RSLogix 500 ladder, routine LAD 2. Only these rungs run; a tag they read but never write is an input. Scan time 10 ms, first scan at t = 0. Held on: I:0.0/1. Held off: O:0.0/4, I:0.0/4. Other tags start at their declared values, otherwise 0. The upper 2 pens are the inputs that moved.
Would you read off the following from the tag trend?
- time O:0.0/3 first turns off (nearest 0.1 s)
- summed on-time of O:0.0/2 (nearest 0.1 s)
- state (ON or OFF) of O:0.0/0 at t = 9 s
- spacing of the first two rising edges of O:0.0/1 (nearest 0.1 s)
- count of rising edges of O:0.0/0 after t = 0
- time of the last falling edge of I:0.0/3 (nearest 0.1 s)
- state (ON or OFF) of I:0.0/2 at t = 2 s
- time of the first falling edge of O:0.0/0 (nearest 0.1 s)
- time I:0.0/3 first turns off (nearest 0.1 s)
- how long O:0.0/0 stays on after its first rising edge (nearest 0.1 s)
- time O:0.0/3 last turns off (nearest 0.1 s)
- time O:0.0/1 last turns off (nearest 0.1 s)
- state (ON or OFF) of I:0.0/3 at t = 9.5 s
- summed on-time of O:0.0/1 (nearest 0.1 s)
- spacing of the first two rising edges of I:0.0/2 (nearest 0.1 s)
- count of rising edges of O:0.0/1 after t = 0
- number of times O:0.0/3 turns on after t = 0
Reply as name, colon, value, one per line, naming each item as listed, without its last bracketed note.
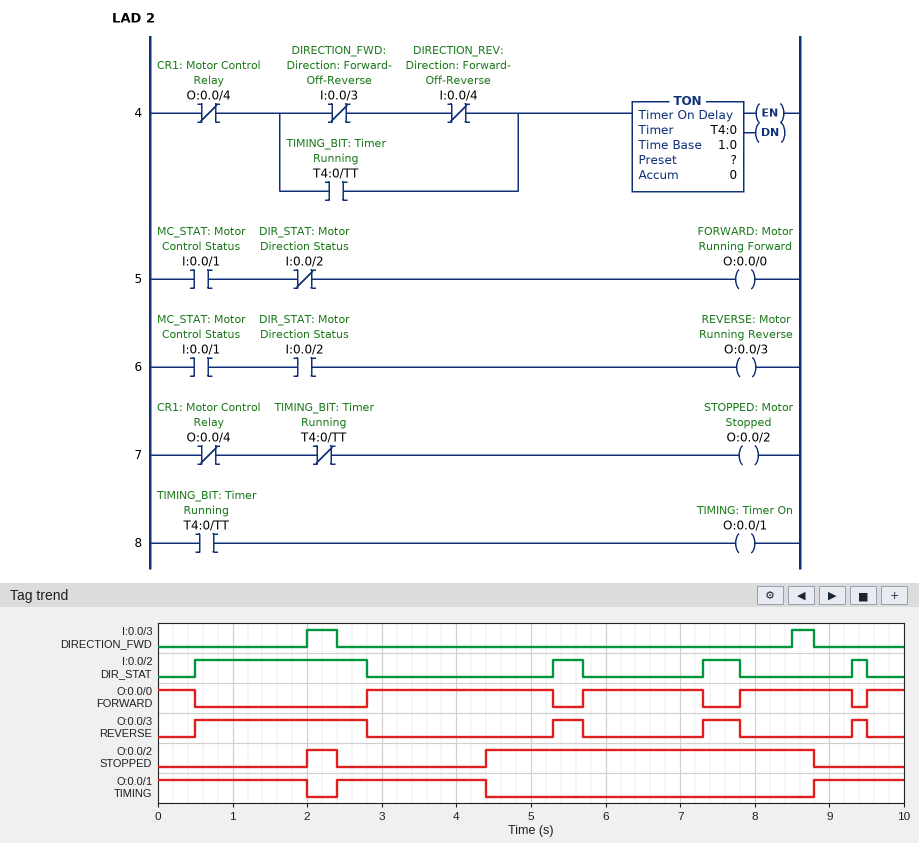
time O:0.0/3 first turns off: 2.8 s
summed on-time of O:0.0/2: 4.8 s
state (ON or OFF) of O:0.0/0 at t = 9 s: ON
spacing of the first two rising edges of O:0.0/1: 6.4 s
count of rising edges of O:0.0/0 after t = 0: 4
time of the last falling edge of I:0.0/3: 8.8 s
state (ON or OFF) of I:0.0/2 at t = 2 s: ON
time of the first falling edge of O:0.0/0: 0.5 s
time I:0.0/3 first turns off: 2.4 s
how long O:0.0/0 stays on after its first rising edge: 2.5 s
time O:0.0/3 last turns off: 9.5 s
time O:0.0/1 last turns off: 4.4 s
state (ON or OFF) of I:0.0/3 at t = 9.5 s: OFF
summed on-time of O:0.0/1: 5.2 s
spacing of the first two rising edges of I:0.0/2: 4.8 s
count of rising edges of O:0.0/1 after t = 0: 2
number of times O:0.0/3 turns on after t = 0: 4
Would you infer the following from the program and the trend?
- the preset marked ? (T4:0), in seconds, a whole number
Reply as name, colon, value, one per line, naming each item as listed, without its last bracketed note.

the preset marked ? (T4:0), in seconds, a whole number: 2 s
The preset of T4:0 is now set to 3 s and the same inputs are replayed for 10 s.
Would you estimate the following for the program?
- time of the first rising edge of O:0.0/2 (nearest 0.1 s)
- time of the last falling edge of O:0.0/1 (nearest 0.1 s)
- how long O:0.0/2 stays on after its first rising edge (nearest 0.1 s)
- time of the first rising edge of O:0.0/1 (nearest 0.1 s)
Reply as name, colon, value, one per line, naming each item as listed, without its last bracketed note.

time of the first rising edge of O:0.0/2: 3.0 s
time of the last falling edge of O:0.0/1: 3.0 s
how long O:0.0/2 stays on after its first rising edge: 5.8 s
time of the first rising edge of O:0.0/1: 8.8 s
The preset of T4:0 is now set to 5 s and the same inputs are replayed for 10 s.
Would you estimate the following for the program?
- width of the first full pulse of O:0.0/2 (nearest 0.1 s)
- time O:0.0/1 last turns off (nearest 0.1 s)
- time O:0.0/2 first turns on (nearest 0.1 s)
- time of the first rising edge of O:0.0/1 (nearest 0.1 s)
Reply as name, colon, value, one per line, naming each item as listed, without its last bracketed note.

width of the first full pulse of O:0.0/2: 3.8 s
time O:0.0/1 last turns off: 5.0 s
time O:0.0/2 first turns on: 5.0 s
time of the first rising edge of O:0.0/1: 8.8 s
